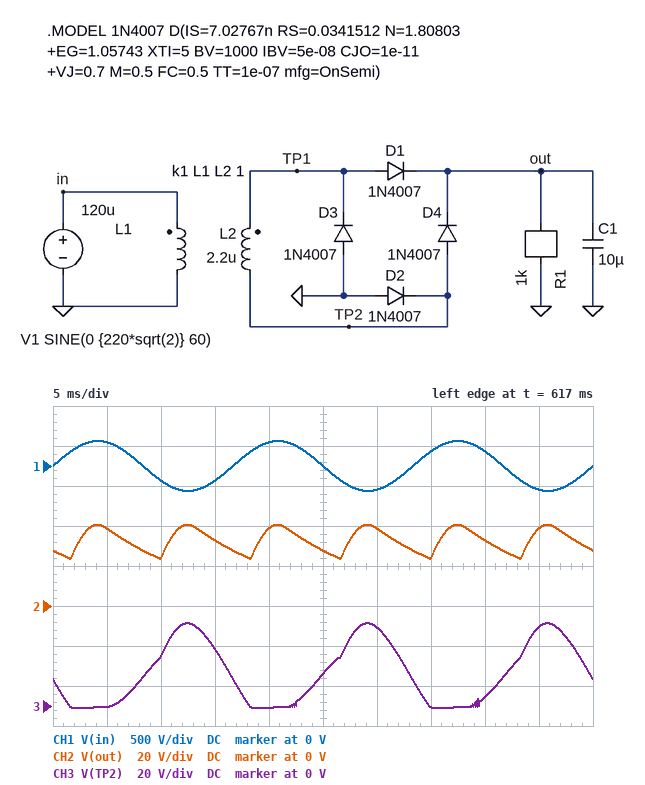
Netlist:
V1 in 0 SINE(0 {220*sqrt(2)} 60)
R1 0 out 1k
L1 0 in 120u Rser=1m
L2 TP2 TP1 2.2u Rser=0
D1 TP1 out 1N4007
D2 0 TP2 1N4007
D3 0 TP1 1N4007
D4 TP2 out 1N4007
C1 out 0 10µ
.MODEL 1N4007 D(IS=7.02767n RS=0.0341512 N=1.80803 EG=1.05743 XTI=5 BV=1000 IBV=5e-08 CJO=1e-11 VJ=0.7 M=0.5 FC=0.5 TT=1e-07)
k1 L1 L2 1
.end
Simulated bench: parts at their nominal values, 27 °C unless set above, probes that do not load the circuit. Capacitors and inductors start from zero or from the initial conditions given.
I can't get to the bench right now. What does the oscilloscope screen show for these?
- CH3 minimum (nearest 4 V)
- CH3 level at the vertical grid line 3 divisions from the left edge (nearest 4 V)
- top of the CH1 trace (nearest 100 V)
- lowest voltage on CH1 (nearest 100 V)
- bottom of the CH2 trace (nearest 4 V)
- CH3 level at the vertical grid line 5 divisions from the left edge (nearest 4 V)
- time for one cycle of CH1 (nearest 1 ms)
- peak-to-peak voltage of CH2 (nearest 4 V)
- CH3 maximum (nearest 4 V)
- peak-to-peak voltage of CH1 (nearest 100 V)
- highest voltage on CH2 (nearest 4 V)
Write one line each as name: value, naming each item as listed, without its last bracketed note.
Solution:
CH3 minimum: 0 V
CH3 level at the vertical grid line 3 divisions from the left edge: 28 V
top of the CH1 trace: 300 V
lowest voltage on CH1: -300 V
bottom of the CH2 trace: 24 V
CH3 level at the vertical grid line 5 divisions from the left edge: 16 V
time for one cycle of CH1: 17 ms
peak-to-peak voltage of CH2: 16 V
CH3 maximum: 40 V
peak-to-peak voltage of CH1: 600 V
highest voltage on CH2: 40 V
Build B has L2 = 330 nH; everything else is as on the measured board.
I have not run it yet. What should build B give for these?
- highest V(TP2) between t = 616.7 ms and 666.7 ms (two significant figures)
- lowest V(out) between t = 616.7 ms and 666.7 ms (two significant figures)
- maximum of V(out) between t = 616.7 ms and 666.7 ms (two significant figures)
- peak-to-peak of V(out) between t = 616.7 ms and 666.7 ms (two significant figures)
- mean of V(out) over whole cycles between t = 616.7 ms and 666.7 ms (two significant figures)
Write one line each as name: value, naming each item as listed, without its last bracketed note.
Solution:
highest V(TP2) between t = 616.7 ms and 666.7 ms: 16 V
lowest V(out) between t = 616.7 ms and 666.7 ms: 8.7 V
maximum of V(out) between t = 616.7 ms and 666.7 ms: 15 V
peak-to-peak of V(out) between t = 616.7 ms and 666.7 ms: 6.3 V
mean of V(out) over whole cycles between t = 616.7 ms and 666.7 ms: 12 V
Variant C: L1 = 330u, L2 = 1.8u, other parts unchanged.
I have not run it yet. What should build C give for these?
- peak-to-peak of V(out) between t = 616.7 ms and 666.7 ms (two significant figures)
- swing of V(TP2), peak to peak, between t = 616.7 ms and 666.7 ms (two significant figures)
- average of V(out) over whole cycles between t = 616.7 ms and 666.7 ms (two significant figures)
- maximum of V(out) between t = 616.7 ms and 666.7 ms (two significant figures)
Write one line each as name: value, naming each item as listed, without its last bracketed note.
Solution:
peak-to-peak of V(out) between t = 616.7 ms and 666.7 ms: 9.1 V
swing of V(TP2), peak to peak, between t = 616.7 ms and 666.7 ms: 23 V
average of V(out) over whole cycles between t = 616.7 ms and 666.7 ms: 17 V
maximum of V(out) between t = 616.7 ms and 666.7 ms: 22 V
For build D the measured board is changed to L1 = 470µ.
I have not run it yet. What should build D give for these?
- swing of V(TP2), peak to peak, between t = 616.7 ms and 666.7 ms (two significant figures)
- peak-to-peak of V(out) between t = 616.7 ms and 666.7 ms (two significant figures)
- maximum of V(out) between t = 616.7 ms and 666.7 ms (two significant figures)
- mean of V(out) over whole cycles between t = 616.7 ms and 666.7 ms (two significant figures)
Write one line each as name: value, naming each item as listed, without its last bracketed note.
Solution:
swing of V(TP2), peak to peak, between t = 616.7 ms and 666.7 ms: 21 V
peak-to-peak of V(out) between t = 616.7 ms and 666.7 ms: 8.4 V
maximum of V(out) between t = 616.7 ms and 666.7 ms: 20 V
mean of V(out) over whole cycles between t = 616.7 ms and 666.7 ms: 16 V
